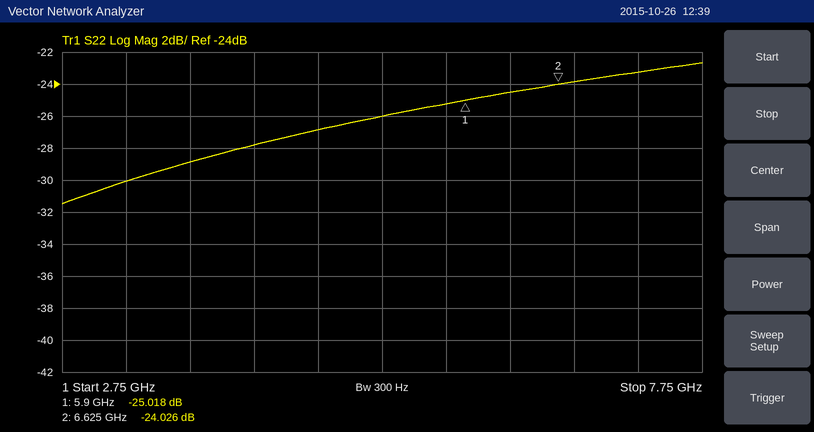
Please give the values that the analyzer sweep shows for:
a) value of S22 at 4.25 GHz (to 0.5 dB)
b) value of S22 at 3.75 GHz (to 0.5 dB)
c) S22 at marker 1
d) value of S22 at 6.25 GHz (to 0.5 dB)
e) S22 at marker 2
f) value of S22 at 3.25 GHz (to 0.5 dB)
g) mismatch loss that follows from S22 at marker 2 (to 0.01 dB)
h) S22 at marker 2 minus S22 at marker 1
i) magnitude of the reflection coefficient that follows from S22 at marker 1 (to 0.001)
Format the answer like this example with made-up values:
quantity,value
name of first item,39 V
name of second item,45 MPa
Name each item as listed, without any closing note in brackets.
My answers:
quantity,value
value of S22 at 4.25 GHz,-28.0 dB
value of S22 at 3.75 GHz,-29.0 dB
S22 at marker 1,-25.018 dB
value of S22 at 6.25 GHz,-24.5 dB
S22 at marker 2,-24.026 dB
value of S22 at 3.25 GHz,-30.0 dB
mismatch loss that follows from S22 at marker 2,0.02 dB
S22 at marker 2 minus S22 at marker 1,0.992 dB
magnitude of the reflection coefficient that follows from S22 at marker 1,0.056
